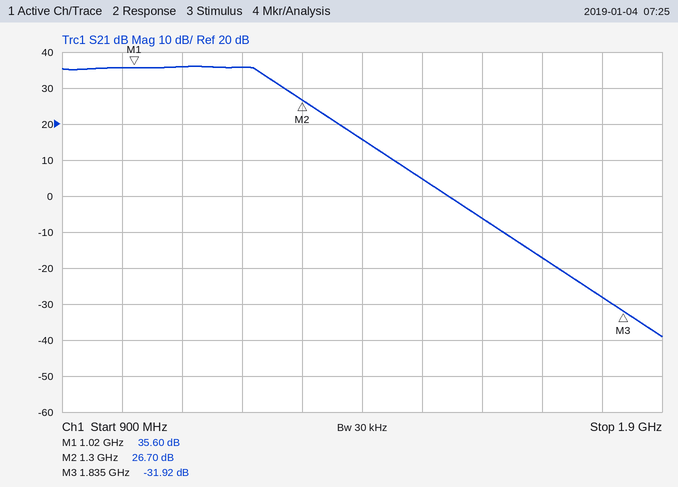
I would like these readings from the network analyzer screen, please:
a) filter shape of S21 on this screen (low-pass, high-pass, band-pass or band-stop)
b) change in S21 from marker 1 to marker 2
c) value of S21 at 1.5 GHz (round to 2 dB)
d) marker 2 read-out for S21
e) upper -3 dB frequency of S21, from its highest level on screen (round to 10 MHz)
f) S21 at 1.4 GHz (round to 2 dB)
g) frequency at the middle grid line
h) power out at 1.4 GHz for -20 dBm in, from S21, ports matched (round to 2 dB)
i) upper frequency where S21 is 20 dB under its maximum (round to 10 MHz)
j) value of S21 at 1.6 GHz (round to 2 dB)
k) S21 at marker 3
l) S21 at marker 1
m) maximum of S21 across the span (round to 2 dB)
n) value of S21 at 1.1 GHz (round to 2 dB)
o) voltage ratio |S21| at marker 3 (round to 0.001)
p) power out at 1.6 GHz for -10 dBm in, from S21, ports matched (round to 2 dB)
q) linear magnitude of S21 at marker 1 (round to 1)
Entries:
low-pass
-8.90 dB
4 dB
26.70 dB
1.24 GHz
16 dB
1.4 GHz
-4 dBm
1.40 GHz
-6 dB
-31.92 dB
35.60 dB
36 dB
36 dB
0.025
-16 dBm
60
